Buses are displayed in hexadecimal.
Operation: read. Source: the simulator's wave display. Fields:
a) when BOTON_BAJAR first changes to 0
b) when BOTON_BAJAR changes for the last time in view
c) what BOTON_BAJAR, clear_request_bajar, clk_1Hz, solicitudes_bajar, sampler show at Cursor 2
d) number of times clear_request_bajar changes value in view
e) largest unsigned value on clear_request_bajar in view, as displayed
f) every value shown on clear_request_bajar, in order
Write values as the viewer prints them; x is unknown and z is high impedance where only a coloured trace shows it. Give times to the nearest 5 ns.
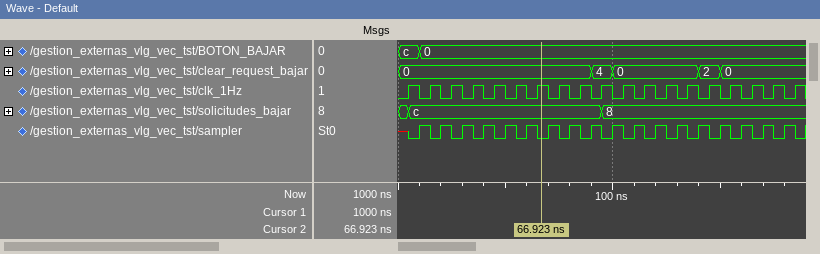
10 ns
10 ns
BOTON_BAJAR=0, clear_request_bajar=0, clk_1Hz=1, solicitudes_bajar=c, sampler=0
4
4
0, 4, 0, 2, 0
